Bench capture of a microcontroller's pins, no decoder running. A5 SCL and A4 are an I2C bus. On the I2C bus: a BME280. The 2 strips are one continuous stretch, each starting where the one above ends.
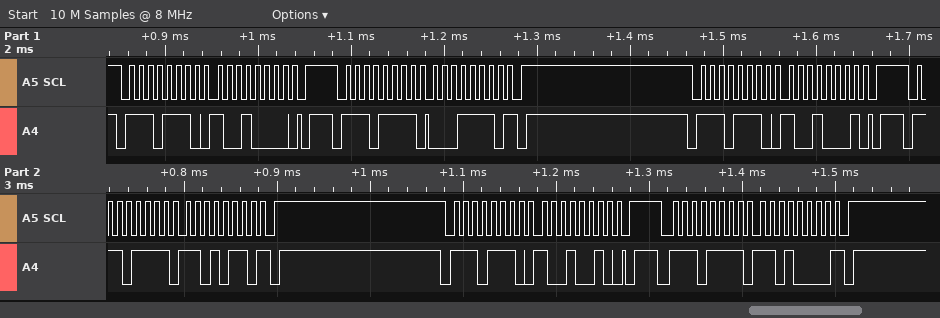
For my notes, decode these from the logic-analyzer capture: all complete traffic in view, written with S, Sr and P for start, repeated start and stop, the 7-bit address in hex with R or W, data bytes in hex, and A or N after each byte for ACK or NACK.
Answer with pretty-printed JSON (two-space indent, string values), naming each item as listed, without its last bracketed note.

{
  "all complete traffic in view, written with S, Sr and P for start, repeated start and stop, the 7-bit address in hex with R or W, data bytes in hex, and A or N after each byte for ACK or NACK": "S 77W A 90 A P S 77R A 1E N P S 77W A 91 A P S 77R A D6 N P S 77W A 92 A P S 77R A D0 N P"
}
